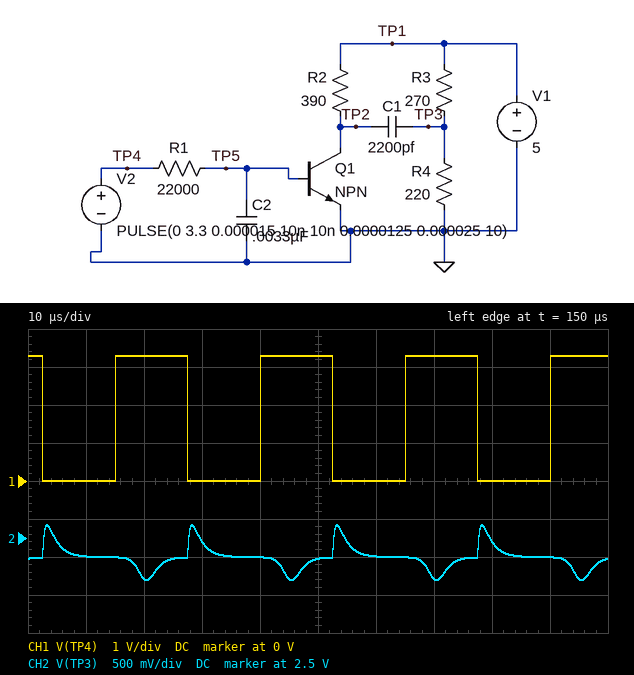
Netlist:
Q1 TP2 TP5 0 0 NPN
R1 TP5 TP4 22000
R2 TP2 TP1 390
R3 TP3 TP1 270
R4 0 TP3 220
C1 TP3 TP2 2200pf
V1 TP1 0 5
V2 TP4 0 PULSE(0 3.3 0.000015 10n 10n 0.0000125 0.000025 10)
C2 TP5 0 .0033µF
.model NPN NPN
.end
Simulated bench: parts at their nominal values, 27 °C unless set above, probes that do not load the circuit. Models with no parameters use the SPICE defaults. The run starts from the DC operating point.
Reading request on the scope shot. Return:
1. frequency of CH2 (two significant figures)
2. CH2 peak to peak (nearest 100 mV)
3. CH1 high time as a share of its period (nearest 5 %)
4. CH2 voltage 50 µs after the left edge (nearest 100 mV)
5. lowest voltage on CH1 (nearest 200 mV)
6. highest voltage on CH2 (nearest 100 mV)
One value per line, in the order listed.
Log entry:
40 kHz
700 mV
50 %
2.2 V
0 V
2.7 V
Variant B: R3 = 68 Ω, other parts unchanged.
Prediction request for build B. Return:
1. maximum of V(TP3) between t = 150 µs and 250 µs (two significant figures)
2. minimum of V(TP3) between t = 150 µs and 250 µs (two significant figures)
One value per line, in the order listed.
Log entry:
4.0 V
3.7 V
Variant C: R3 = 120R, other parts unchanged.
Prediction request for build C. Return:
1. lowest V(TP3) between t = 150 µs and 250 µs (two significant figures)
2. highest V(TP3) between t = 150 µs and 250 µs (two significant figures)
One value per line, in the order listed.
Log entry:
3.0 V
3.5 V
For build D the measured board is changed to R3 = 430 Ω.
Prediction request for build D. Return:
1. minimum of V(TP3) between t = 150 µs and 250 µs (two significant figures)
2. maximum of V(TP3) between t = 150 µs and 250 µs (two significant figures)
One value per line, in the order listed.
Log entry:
1.3 V
2.2 V
